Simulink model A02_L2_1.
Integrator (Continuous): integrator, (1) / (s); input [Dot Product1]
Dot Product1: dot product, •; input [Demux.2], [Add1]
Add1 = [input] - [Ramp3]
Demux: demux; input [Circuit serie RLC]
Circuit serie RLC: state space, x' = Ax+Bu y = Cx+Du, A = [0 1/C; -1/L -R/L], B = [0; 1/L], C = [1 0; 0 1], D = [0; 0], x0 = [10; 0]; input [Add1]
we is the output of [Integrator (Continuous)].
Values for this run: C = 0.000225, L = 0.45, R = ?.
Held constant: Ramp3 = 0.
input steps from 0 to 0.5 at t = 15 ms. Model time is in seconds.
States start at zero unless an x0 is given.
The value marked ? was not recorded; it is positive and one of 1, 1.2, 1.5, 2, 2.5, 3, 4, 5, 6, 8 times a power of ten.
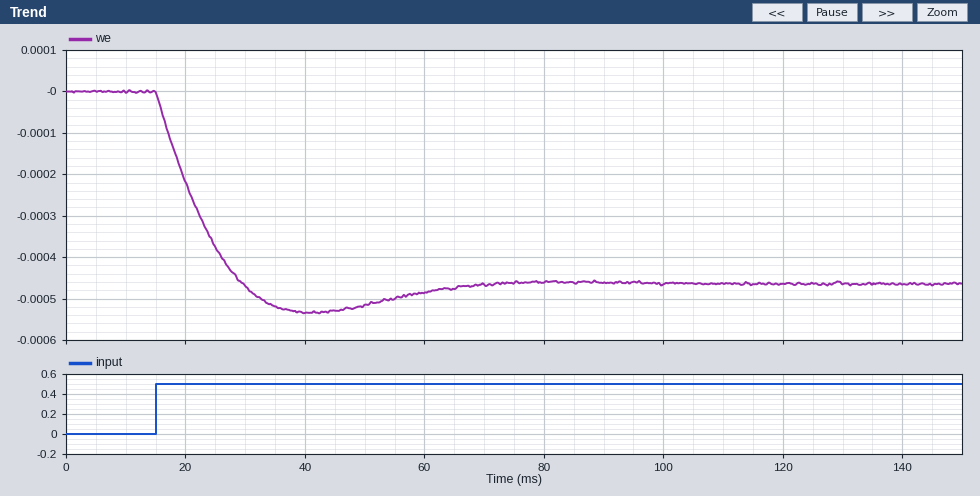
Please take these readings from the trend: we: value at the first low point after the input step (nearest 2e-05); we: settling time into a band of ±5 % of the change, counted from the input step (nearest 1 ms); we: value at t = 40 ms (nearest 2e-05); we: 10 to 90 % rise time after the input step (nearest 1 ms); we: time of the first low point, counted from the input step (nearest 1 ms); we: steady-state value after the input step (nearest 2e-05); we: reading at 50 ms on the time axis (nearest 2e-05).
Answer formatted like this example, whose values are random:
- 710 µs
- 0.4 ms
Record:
- -0.00054
- 44 ms
- -0.00054
- 11 ms
- 26 ms
- -0.00046
- -0.00052
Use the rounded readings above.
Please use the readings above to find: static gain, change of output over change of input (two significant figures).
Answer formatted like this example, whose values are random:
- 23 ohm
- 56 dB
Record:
- -0.00092
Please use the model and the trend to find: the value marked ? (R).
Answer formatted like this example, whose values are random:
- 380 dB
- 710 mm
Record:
- 60
